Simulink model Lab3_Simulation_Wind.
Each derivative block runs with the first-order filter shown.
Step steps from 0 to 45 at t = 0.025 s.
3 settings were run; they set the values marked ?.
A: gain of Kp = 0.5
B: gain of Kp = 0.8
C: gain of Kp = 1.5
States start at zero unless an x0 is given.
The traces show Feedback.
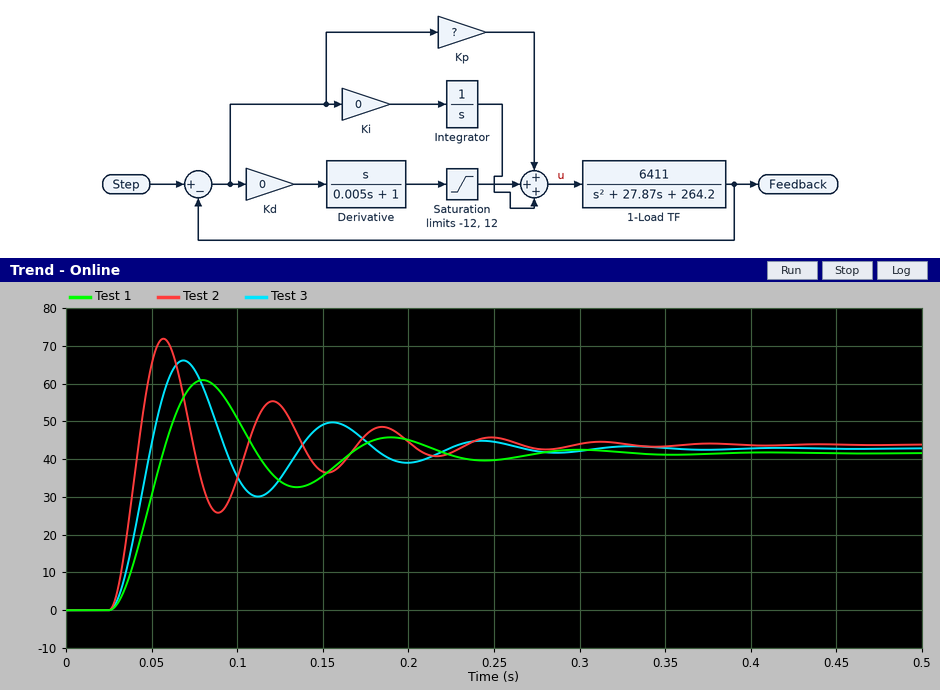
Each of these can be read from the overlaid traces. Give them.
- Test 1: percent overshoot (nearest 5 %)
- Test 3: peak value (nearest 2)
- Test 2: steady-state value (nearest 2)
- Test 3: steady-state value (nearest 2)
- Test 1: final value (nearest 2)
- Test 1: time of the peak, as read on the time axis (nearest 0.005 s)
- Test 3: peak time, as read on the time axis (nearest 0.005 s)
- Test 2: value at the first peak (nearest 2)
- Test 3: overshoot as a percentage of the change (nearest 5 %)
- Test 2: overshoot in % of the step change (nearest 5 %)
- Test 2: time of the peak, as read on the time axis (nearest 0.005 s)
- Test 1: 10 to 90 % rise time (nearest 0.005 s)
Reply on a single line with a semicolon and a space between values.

45 %; 66; 44; 42; 42; 0.080 s; 0.070 s; 72; 55 %; 65 %; 0.055 s; 0.020 s
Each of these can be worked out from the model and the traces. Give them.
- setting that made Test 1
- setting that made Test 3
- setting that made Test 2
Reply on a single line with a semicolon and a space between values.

A; B; C
